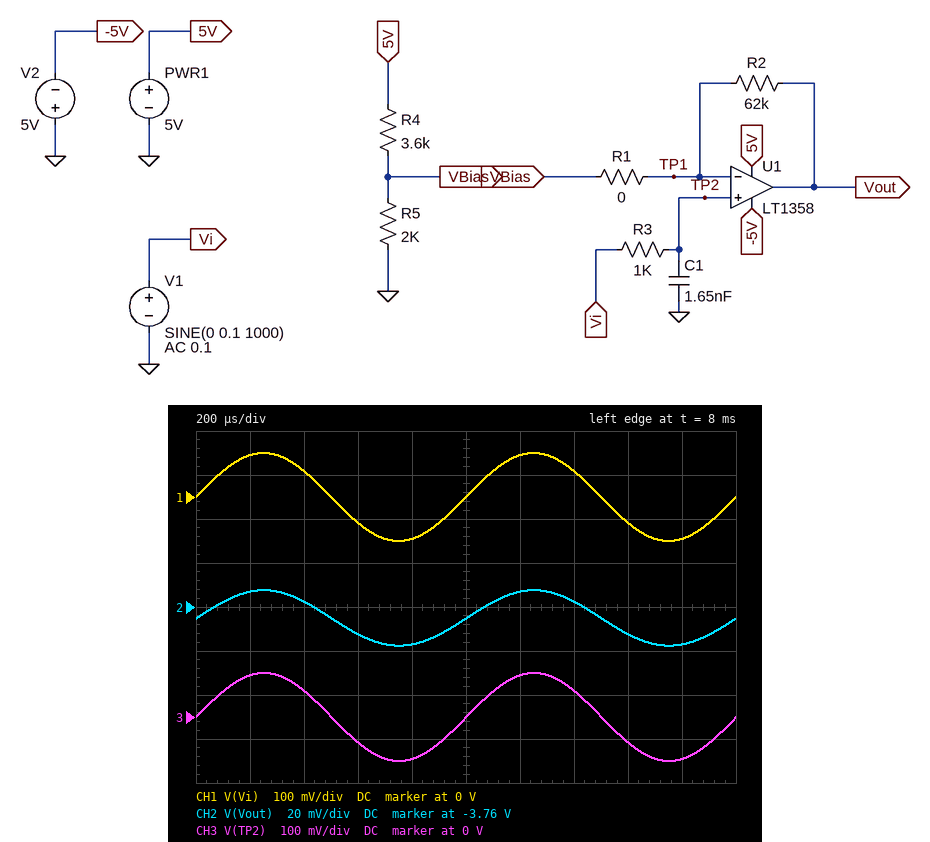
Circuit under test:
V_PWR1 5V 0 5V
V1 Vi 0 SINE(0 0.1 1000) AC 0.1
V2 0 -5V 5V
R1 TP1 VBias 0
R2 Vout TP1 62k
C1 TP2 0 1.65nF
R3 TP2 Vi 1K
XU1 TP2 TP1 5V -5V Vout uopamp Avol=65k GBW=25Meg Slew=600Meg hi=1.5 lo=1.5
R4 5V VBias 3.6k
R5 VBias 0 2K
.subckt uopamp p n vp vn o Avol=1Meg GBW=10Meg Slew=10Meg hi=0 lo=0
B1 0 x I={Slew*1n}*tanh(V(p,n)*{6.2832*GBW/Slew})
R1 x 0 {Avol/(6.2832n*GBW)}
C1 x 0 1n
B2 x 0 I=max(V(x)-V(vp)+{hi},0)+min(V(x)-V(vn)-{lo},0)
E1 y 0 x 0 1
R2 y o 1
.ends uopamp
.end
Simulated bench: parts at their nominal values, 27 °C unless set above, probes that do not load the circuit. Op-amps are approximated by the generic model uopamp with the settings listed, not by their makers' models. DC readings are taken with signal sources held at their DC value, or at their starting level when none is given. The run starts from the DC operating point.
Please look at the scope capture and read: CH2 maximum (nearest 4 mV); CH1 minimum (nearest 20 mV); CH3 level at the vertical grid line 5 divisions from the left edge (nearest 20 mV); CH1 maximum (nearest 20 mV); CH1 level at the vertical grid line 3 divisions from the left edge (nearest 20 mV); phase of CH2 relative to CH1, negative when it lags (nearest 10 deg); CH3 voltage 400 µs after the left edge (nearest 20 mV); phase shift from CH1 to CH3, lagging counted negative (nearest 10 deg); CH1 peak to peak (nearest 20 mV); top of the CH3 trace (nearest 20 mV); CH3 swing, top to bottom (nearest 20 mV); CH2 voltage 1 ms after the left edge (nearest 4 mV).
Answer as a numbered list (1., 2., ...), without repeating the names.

1. -3.752 V
2. -100 mV
3. 0 V
4. 100 mV
5. -60 mV
6. 0 deg
7. 60 mV
8. 0 deg
9. 200 mV
10. 100 mV
11. 200 mV
12. -3.764 V
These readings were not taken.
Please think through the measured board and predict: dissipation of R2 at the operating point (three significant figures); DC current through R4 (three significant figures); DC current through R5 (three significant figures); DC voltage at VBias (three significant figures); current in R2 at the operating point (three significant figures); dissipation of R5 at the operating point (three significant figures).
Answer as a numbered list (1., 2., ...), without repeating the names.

1. 502 µW
2. 885 µA
3. 907 µA
4. 1.81 V
5. 90.0 µA
6. 1.64 mW
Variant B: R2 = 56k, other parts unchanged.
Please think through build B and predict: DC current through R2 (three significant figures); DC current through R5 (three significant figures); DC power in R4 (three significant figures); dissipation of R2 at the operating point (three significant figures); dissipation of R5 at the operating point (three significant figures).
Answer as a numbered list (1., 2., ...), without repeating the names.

1. 99.4 µA
2. 902 µA
3. 2.84 mW
4. 554 µW
5. 1.63 mW
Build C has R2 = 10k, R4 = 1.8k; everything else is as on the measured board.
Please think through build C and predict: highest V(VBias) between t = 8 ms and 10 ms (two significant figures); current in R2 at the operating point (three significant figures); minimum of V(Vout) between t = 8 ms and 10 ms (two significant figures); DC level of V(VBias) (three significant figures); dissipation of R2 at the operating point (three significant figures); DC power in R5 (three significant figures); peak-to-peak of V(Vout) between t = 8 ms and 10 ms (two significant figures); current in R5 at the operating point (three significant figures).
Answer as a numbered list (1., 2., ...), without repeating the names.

1. 2.2 V
2. 599 µA
3. -3.8 V
4. 2.18 V
5. 3.59 mW
6. 2.38 mW
7. 23 mV
8. 1.09 mA
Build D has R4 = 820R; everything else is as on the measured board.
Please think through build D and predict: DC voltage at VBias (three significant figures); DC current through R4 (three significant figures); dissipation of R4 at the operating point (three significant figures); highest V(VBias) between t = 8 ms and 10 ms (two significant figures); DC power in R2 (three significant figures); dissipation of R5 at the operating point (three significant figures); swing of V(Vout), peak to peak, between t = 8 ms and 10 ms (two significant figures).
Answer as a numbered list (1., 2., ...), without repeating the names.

1. 3.53 V
2. 1.79 mA
3. 2.63 mW
4. 3.5 V
5. 899 µW
6. 6.23 mW
7. 15 mV
